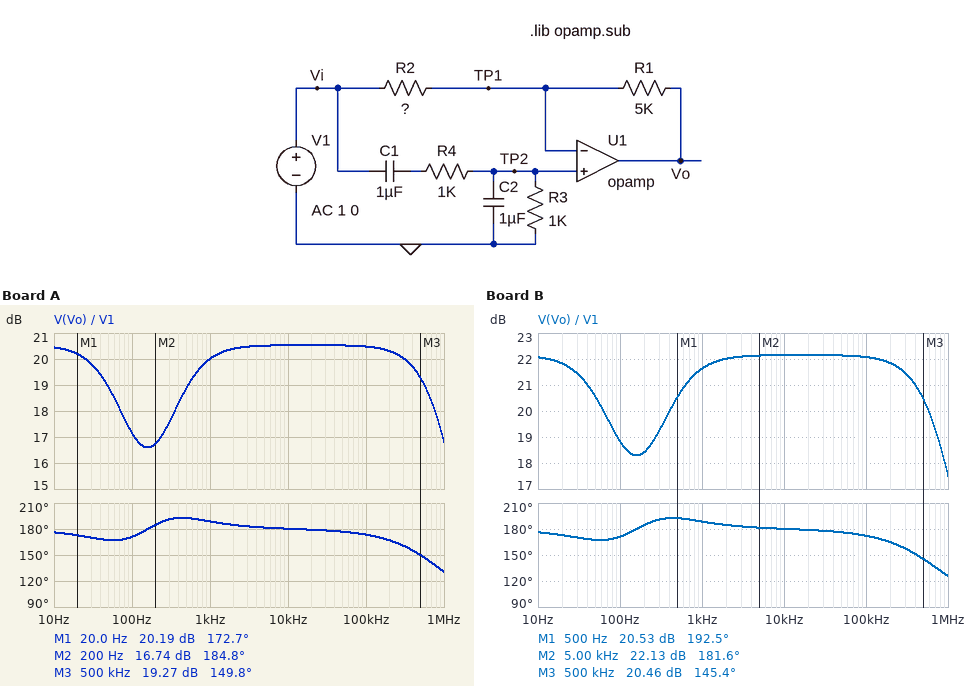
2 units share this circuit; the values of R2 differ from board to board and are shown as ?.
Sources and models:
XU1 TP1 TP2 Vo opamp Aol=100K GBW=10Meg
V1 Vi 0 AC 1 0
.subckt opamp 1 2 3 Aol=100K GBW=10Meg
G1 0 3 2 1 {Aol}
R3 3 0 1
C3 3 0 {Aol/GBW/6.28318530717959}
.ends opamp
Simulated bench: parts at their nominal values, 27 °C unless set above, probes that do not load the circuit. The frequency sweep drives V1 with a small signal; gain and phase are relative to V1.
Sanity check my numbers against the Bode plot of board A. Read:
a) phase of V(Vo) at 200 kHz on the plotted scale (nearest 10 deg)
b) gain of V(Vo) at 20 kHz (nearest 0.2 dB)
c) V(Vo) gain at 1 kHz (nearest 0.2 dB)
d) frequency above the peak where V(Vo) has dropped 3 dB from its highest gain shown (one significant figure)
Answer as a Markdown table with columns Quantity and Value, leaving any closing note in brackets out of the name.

| Quantity | Value |
|---|---|
| phase of V(Vo) at 200 kHz on the plotted scale | 170 deg |
| gain of V(Vo) at 20 kHz | 20.6 dB |
| V(Vo) gain at 1 kHz | 20.0 dB |
| frequency above the peak where V(Vo) has dropped 3 dB from its highest gain shown | 900 kHz |
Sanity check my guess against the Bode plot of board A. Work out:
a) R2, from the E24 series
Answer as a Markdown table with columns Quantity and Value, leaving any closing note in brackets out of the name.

| Quantity | Value |
|---|---|
| R2, from the E24 series | 470 Ω |
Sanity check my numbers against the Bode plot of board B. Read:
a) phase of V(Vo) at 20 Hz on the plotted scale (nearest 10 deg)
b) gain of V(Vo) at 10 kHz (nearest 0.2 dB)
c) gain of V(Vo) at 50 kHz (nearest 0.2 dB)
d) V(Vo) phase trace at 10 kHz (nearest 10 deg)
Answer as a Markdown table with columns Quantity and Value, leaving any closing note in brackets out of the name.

| Quantity | Value |
|---|---|
| phase of V(Vo) at 20 Hz on the plotted scale | 170 deg |
| gain of V(Vo) at 10 kHz | 22.2 dB |
| gain of V(Vo) at 50 kHz | 22.2 dB |
| V(Vo) phase trace at 10 kHz | 180 deg |
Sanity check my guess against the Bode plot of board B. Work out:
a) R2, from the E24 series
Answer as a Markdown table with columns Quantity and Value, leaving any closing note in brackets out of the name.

| Quantity | Value |
|---|---|
| R2, from the E24 series | 390 Ω |
